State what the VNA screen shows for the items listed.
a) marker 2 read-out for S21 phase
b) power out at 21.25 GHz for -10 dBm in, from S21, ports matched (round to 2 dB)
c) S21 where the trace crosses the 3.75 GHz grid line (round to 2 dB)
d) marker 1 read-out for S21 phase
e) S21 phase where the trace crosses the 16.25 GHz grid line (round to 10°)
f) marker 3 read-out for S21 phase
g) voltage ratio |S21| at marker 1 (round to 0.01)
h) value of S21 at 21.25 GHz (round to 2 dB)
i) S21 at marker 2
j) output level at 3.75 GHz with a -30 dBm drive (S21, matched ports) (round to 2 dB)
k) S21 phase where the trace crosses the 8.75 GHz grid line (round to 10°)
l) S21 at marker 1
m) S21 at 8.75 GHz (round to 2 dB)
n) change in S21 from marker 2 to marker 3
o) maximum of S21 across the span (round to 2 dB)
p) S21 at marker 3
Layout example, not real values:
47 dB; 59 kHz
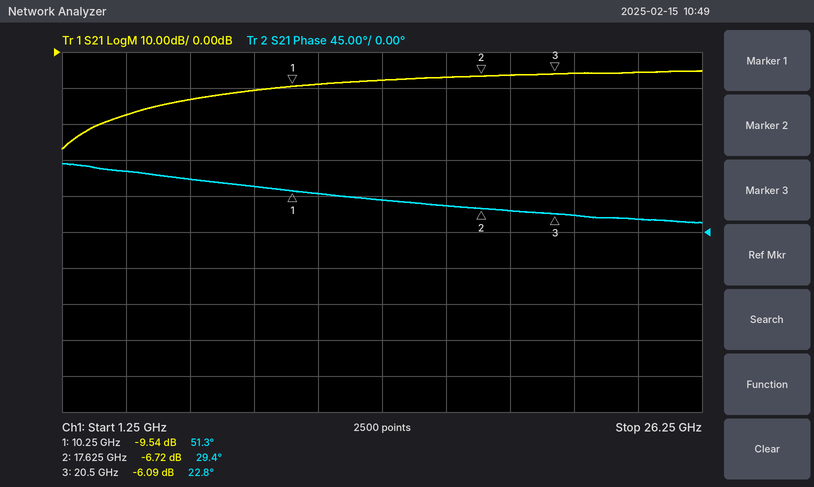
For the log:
29.4°; -16 dBm; -18 dB; 51.3°; 30°; 22.8°; 0.33; -6 dB; -6.72 dB; -48 dBm; 60°; -9.54 dB; -10 dB; 0.63 dB; -6 dB; -6.09 dB
